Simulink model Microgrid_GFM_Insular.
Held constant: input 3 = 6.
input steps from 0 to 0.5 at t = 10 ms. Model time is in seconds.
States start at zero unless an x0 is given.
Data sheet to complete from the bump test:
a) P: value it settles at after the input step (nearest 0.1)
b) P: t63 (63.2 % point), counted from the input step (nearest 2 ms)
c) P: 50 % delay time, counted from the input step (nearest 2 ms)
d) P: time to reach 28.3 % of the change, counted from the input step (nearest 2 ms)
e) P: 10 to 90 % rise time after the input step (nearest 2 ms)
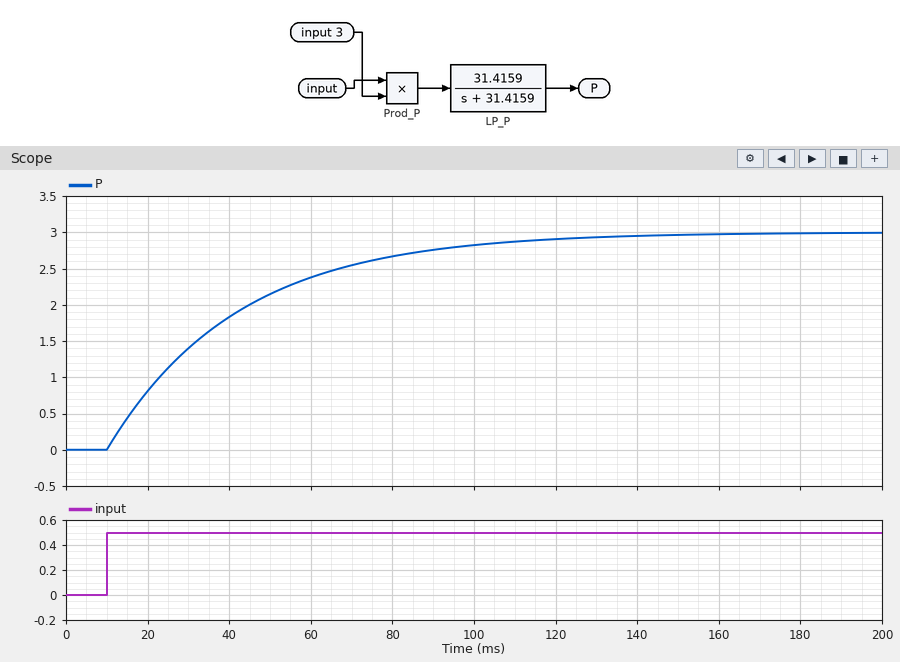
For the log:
3.0
32 ms
22 ms
10 ms
70 ms
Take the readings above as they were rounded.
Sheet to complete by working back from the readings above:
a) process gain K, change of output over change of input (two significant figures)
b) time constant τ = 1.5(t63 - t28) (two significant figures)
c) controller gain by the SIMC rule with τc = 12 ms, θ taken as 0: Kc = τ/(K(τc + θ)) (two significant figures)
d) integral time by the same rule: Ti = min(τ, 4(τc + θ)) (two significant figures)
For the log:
6.0
33 ms
0.46
33 ms
